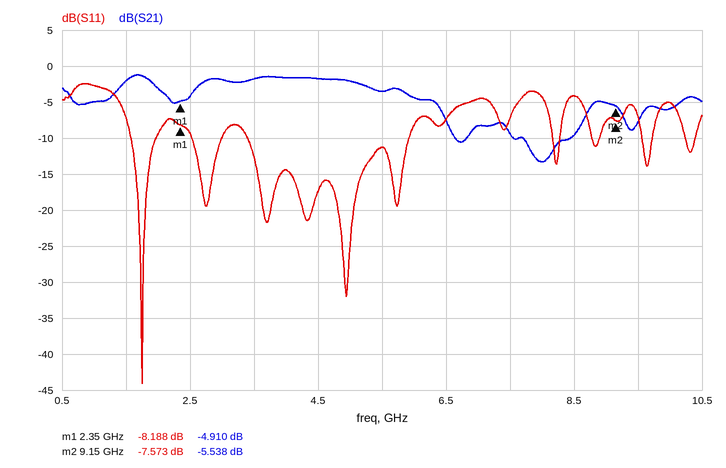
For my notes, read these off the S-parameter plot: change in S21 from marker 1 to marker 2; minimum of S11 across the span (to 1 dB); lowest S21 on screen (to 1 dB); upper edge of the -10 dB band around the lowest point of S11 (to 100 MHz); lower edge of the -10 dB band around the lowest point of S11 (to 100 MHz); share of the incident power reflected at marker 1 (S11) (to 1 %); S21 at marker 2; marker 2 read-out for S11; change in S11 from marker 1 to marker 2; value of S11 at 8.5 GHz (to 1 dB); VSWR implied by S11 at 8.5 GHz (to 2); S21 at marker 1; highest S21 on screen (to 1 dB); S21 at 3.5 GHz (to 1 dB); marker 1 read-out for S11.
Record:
-0.628 dB
-44 dB
-13 dB
2.0 GHz
1.6 GHz
15 %
-5.538 dB
-7.573 dB
0.615 dB
-4 dB
4
-4.910 dB
-1 dB
-2 dB
-8.188 dB
